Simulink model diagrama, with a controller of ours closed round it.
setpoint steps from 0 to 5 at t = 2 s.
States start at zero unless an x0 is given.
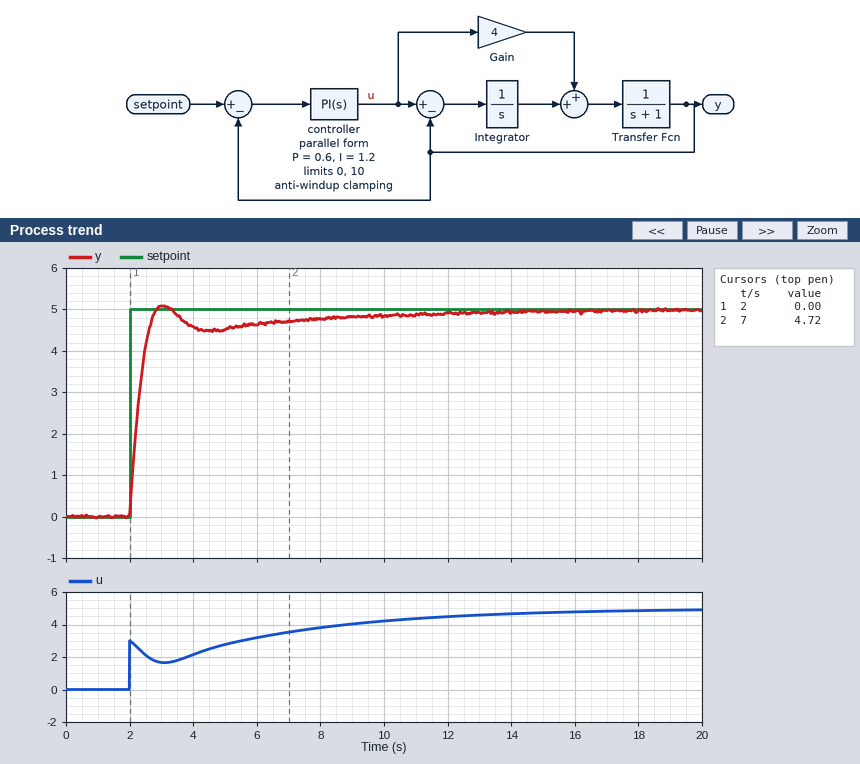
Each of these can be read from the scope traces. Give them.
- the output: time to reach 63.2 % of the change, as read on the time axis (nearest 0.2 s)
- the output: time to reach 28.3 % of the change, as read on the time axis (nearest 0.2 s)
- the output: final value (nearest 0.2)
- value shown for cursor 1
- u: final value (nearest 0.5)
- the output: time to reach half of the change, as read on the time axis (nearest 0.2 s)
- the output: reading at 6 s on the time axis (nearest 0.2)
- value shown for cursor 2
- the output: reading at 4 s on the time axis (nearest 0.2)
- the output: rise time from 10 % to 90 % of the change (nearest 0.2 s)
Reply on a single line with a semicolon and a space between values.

2.4 s; 2.2 s; 5.0; 0.00; 5.0; 2.2 s; 4.6; 4.72; 4.6; 0.6 s
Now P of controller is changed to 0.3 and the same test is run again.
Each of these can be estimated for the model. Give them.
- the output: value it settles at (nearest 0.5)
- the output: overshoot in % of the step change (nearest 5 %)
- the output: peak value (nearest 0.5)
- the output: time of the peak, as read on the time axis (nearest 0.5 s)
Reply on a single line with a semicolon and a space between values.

5.0; 10 %; 5.5; 3.0 s
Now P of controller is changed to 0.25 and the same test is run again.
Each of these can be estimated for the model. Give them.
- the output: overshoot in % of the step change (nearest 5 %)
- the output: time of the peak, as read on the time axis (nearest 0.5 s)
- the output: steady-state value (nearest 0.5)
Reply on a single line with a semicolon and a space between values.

15 %; 3.0 s; 5.0
